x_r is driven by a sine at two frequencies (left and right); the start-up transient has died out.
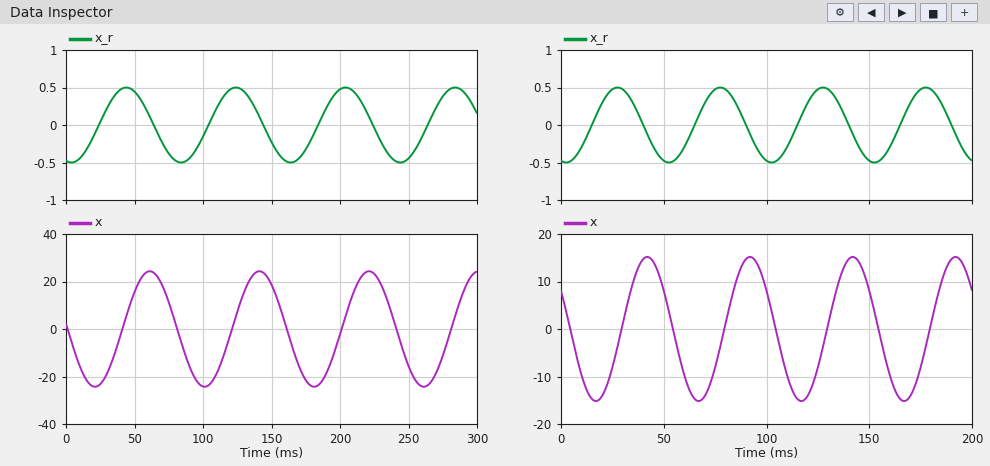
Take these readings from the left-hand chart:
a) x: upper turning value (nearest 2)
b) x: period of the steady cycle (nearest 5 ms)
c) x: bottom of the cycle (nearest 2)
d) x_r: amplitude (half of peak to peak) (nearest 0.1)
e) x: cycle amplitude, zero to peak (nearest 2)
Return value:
24
80 ms
-24
0.5
24
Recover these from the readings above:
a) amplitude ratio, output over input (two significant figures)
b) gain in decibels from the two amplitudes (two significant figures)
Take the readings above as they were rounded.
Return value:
48
34 dB
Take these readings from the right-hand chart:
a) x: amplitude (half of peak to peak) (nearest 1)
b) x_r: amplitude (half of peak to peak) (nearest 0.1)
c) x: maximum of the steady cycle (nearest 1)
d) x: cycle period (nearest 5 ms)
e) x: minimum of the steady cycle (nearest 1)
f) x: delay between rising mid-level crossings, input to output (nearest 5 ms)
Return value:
15
0.5
15
50 ms
-15
15 ms
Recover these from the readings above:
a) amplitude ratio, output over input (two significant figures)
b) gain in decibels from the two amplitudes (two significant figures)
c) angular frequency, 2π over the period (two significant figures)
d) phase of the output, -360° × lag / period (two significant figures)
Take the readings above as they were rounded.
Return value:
30
30 dB
0.13 rad/ms
-110°
